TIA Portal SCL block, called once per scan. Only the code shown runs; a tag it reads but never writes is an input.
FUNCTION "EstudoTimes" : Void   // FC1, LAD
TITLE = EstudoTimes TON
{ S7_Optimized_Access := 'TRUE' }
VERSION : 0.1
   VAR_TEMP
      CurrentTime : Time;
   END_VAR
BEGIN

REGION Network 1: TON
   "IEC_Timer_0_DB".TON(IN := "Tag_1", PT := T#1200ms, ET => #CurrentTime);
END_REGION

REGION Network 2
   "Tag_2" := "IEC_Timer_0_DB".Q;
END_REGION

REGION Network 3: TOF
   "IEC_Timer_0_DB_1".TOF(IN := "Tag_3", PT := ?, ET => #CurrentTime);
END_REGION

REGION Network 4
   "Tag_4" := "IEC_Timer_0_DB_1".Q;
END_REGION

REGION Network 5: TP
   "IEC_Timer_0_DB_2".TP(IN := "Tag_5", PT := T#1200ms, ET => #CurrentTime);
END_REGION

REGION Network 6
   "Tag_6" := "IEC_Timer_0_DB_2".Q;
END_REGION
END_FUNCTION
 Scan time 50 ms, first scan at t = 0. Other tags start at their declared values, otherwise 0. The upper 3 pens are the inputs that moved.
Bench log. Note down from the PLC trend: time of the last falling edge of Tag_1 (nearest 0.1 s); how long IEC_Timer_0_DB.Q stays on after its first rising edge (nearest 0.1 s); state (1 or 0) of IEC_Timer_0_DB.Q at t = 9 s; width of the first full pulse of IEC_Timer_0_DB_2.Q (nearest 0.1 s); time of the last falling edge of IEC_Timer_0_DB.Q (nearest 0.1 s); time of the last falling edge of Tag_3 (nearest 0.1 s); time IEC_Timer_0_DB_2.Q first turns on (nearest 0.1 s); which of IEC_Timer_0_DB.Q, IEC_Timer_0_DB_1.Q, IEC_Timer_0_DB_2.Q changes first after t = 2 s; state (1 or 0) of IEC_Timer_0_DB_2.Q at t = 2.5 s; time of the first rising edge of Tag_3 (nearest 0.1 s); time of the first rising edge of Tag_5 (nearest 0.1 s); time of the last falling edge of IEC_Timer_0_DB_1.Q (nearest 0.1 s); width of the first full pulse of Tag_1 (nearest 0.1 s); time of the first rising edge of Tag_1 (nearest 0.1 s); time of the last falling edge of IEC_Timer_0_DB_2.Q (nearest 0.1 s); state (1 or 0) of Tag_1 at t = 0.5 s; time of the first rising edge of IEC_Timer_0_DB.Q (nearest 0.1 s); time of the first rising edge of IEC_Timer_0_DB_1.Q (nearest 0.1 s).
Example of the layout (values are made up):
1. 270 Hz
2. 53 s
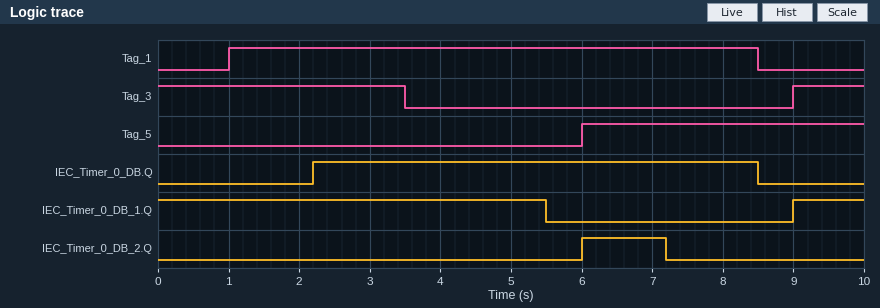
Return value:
1. 8.5 s
2. 6.3 s
3. 0
4. 1.2 s
5. 8.5 s
6. 3.5 s
7. 6.0 s
8. IEC_Timer_0_DB.Q
9. 0
10. 9.0 s
11. 6.0 s
12. 5.5 s
13. 7.5 s
14. 1.0 s
15. 7.2 s
16. 0
17. 2.2 s
18. 9.0 s
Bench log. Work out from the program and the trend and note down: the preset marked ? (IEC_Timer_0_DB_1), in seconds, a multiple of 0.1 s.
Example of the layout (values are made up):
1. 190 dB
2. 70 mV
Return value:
1. 2.0 s
